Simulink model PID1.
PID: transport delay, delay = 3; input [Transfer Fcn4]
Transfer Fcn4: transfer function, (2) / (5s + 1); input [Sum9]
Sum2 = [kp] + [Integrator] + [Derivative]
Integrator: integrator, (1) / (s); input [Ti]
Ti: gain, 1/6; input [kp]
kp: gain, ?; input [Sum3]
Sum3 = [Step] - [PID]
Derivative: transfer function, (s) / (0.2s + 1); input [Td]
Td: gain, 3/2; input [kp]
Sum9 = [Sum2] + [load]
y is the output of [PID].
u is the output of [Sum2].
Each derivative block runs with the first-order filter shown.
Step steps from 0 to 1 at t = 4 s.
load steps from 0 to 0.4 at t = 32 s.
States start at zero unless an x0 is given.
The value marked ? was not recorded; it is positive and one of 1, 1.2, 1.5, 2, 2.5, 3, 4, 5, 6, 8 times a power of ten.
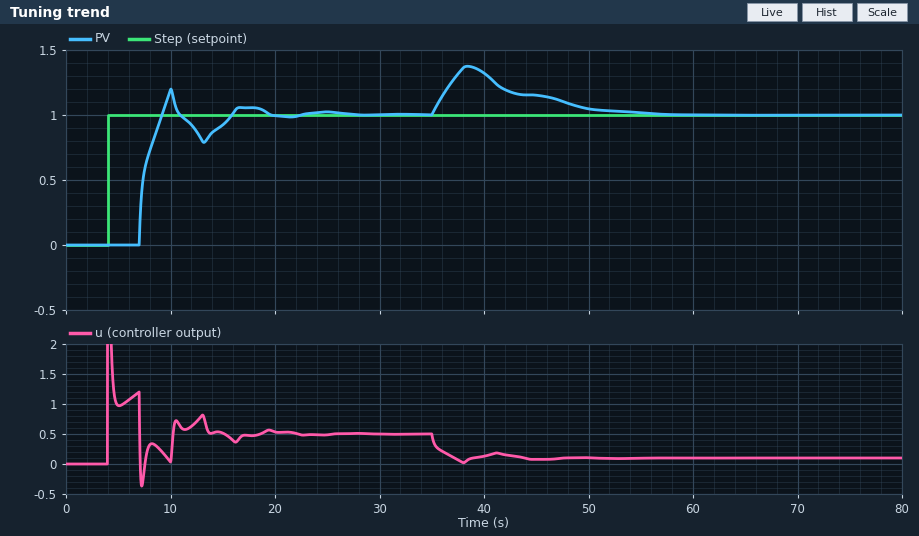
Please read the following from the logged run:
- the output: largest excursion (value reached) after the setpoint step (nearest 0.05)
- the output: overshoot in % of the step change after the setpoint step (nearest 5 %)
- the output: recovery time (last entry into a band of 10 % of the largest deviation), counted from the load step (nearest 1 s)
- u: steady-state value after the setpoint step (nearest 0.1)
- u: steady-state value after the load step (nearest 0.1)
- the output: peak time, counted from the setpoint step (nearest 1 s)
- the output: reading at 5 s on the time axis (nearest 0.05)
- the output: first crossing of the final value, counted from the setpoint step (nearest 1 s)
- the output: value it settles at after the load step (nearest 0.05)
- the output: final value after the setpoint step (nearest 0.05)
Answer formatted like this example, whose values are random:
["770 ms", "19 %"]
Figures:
["1.20", "20 %", "19 s", "0.5", "0.1", "6 s", "0.00", "5 s", "1.00", "1.00"]
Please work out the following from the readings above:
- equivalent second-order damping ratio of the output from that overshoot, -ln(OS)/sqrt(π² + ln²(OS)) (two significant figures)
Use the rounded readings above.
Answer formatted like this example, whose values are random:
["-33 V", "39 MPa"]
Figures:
["0.46"]
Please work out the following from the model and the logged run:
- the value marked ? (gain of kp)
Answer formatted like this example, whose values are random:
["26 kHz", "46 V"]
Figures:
["0.8"]
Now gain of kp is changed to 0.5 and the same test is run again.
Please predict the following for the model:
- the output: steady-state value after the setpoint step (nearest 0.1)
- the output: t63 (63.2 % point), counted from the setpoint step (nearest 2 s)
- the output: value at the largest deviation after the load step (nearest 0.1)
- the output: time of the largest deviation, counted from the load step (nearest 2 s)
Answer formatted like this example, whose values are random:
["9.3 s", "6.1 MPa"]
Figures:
["1.0", "6 s", "1.4", "8 s"]
